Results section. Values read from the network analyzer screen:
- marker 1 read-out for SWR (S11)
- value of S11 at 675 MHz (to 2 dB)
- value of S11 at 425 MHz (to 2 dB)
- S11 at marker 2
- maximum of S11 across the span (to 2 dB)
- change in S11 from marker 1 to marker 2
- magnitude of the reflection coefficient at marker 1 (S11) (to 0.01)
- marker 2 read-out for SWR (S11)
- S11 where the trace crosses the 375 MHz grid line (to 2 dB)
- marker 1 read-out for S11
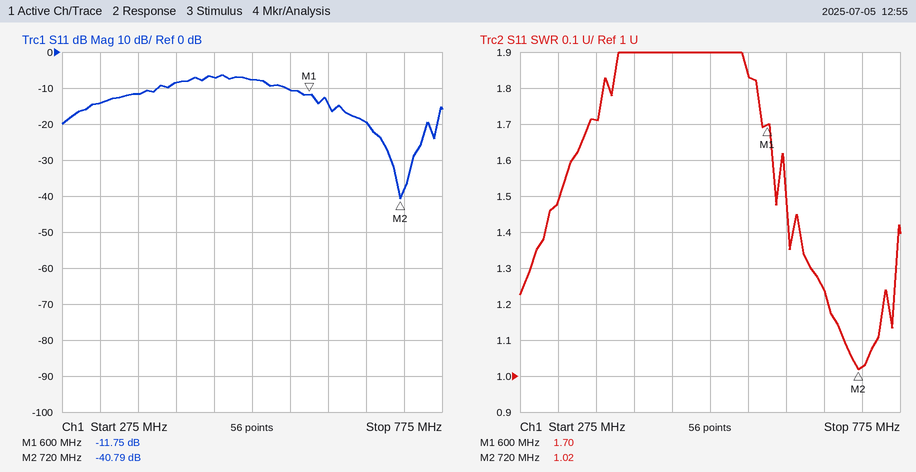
1.70
-20 dB
-8 dB
-40.79 dB
-6 dB
-29.04 dB
0.26
1.02
-12 dB
-11.75 dB
